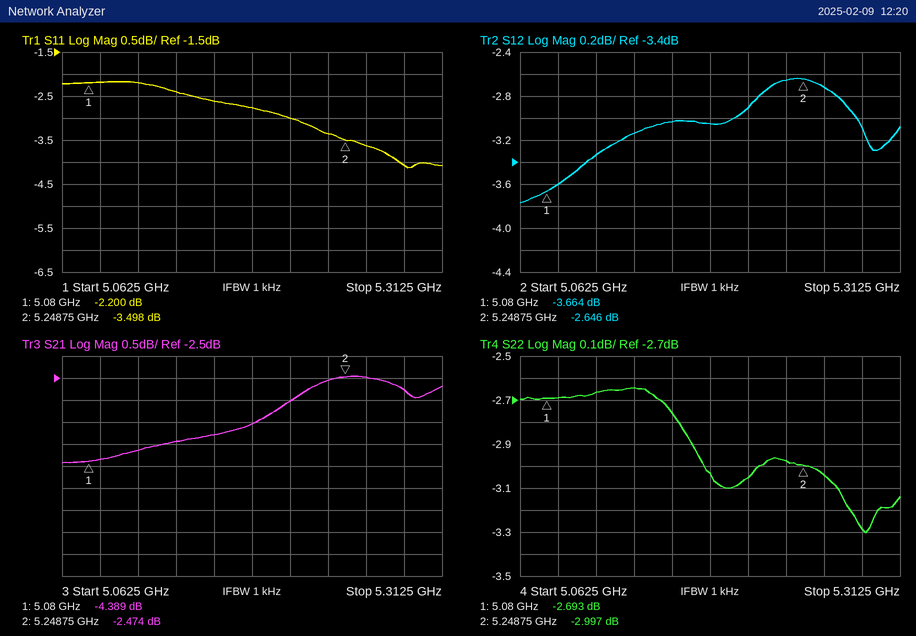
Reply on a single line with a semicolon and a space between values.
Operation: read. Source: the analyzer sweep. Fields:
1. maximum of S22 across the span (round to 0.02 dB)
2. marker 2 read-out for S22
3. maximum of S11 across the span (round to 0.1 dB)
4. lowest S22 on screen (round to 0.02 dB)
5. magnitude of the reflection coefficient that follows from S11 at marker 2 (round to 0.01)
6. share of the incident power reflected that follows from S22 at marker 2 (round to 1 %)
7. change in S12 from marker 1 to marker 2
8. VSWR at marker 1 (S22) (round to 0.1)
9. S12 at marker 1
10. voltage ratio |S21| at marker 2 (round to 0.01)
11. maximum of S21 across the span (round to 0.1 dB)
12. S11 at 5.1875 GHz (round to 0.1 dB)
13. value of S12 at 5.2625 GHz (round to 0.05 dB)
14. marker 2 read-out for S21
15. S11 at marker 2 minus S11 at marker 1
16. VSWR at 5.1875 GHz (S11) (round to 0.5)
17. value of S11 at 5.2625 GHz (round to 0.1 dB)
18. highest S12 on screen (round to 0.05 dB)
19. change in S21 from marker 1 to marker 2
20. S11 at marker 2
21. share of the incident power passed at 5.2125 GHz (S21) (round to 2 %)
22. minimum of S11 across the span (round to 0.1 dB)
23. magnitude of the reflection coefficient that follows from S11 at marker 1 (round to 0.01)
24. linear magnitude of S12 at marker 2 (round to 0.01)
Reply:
-2.64 dB; -2.997 dB; -2.2 dB; -3.30 dB; 0.67; 50 %; 1.018 dB; 6.5; -3.664 dB; 0.75; -2.5 dB; -2.8 dB; -2.70 dB; -2.474 dB; -1.298 dB; 6.5; -3.6 dB; -2.65 dB; 1.915 dB; -3.498 dB; 50 %; -4.1 dB; 0.78; 0.74
